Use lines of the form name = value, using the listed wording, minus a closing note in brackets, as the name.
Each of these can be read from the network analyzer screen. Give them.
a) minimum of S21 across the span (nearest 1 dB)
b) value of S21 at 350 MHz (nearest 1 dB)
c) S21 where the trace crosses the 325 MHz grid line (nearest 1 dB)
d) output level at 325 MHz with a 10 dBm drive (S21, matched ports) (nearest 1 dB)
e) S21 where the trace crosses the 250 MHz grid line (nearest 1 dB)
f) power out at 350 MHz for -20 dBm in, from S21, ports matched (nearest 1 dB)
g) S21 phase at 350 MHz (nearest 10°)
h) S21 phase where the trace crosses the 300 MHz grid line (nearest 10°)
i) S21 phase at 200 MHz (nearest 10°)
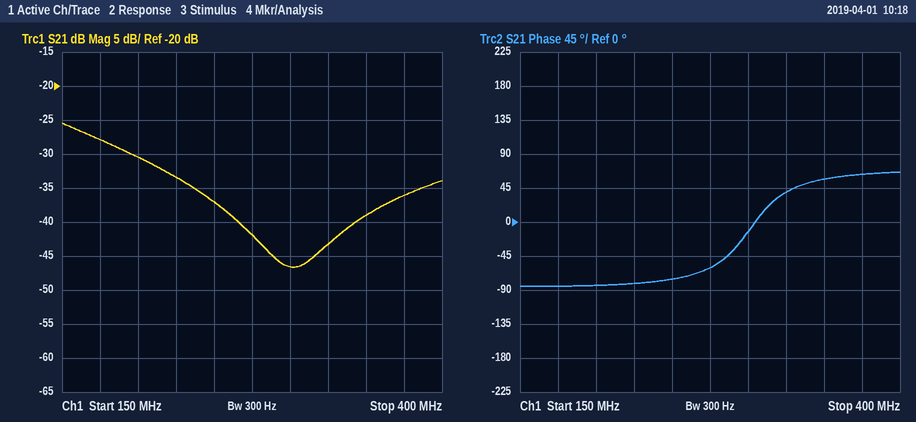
minimum of S21 across the span = -47 dB
value of S21 at 350 MHz = -39 dB
S21 where the trace crosses the 325 MHz grid line = -43 dB
output level at 325 MHz with a 10 dBm drive (S21, matched ports) = -33 dBm
S21 where the trace crosses the 250 MHz grid line = -37 dB
power out at 350 MHz for -20 dBm in, from S21, ports matched = -59 dBm
S21 phase at 350 MHz = 60°
S21 phase where the trace crosses the 300 MHz grid line = -10°
S21 phase at 200 MHz = -80°
